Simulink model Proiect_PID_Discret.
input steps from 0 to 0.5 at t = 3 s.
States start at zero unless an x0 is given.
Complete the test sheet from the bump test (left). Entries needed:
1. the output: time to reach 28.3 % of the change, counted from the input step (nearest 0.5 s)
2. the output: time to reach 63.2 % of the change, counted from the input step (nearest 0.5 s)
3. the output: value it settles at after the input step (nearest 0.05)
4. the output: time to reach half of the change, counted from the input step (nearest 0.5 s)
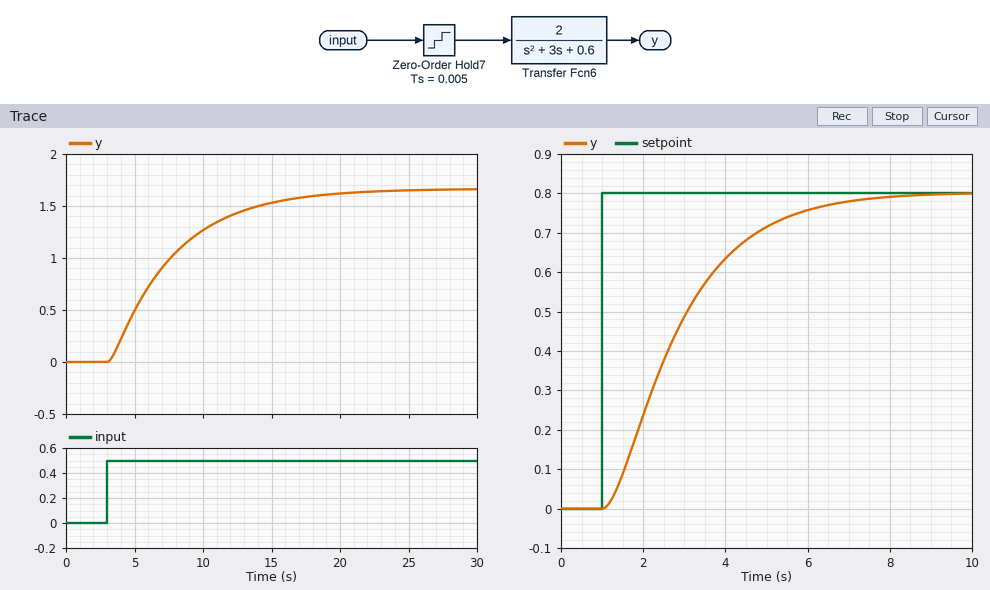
2.0 s
5.0 s
1.65
3.5 s
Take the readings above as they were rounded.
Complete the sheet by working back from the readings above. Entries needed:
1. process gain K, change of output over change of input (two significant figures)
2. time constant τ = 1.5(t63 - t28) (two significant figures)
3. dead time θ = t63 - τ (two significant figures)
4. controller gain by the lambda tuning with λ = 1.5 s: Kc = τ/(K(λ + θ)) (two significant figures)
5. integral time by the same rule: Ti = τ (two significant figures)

3.3
4.5 s
0.50 s
0.68
4.5 s
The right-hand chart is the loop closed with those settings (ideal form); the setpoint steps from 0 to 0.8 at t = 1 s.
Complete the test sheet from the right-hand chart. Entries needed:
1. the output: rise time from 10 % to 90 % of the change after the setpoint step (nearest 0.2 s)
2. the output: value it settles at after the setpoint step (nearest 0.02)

3.6 s
0.80
